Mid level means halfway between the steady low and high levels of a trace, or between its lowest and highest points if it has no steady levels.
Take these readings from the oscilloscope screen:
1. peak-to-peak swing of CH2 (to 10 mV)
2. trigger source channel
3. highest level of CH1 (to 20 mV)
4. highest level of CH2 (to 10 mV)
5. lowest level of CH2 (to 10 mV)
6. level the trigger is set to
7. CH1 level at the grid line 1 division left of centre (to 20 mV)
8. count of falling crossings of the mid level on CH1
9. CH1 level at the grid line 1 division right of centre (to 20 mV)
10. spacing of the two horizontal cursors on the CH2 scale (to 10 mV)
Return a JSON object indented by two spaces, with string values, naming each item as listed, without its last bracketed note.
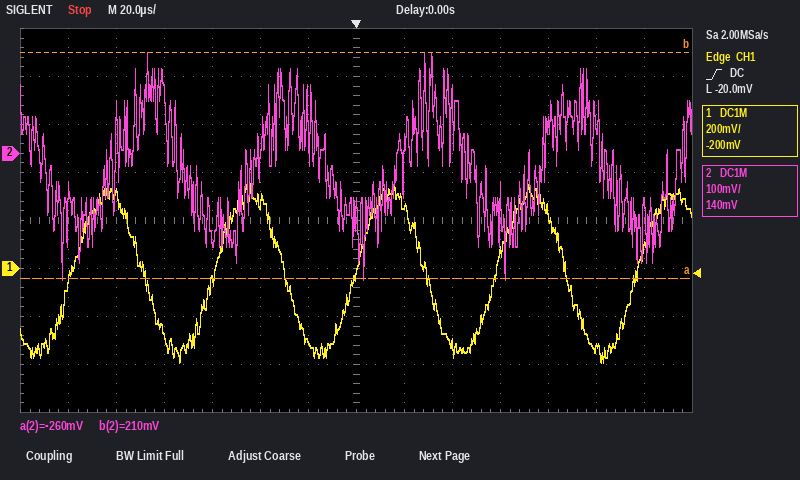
{
  "peak-to-peak swing of CH2": "470 mV",
  "trigger source channel": "CH1",
  "highest level of CH1": "360 mV",
  "highest level of CH2": "210 mV",
  "lowest level of CH2": "-260 mV",
  "level the trigger is set to": "-20.0 mV",
  "CH1 level at the grid line 1 division left of centre": "-300 mV",
  "count of falling crossings of the mid level on CH1": "4",
  "CH1 level at the grid line 1 division right of centre": "260 mV",
  "spacing of the two horizontal cursors on the CH2 scale": "470 mV"
}
